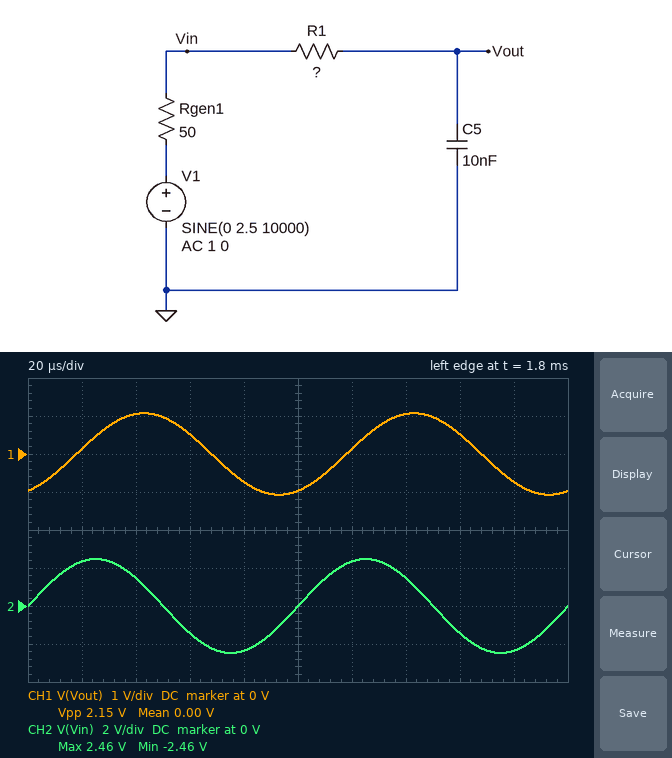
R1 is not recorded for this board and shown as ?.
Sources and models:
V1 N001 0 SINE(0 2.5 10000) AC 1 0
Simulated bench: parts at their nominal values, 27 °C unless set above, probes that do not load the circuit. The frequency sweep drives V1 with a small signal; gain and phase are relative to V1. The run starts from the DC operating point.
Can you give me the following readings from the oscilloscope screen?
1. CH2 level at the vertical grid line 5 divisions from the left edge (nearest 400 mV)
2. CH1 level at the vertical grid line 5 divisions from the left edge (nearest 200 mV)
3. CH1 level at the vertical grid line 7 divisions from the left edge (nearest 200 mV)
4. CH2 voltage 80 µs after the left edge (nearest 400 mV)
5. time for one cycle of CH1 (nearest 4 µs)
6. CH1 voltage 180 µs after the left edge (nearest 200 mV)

0 V
-1.0 V
1.0 V
-2.4 V
100 µs
-800 mV
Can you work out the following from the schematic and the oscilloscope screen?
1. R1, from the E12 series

3.3 kΩ
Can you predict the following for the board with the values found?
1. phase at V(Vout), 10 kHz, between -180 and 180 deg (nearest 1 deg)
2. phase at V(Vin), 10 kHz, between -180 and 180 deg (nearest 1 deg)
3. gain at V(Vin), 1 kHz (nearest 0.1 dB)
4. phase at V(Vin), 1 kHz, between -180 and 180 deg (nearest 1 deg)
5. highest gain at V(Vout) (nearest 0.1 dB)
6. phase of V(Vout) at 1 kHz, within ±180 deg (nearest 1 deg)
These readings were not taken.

-65 deg
0 deg
0 dB
0 deg
0 dB
-12 deg
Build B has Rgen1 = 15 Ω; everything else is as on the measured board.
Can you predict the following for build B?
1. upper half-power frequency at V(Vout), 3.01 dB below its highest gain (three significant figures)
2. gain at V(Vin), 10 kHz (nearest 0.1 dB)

4.80 kHz
0 dB
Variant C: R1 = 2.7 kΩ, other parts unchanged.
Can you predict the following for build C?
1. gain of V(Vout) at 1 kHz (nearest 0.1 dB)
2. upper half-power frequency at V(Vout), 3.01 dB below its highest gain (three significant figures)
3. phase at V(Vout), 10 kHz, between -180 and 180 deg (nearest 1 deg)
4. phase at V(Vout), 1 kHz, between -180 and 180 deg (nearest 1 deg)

-0.1 dB
5.79 kHz
-60 deg
-10 deg
